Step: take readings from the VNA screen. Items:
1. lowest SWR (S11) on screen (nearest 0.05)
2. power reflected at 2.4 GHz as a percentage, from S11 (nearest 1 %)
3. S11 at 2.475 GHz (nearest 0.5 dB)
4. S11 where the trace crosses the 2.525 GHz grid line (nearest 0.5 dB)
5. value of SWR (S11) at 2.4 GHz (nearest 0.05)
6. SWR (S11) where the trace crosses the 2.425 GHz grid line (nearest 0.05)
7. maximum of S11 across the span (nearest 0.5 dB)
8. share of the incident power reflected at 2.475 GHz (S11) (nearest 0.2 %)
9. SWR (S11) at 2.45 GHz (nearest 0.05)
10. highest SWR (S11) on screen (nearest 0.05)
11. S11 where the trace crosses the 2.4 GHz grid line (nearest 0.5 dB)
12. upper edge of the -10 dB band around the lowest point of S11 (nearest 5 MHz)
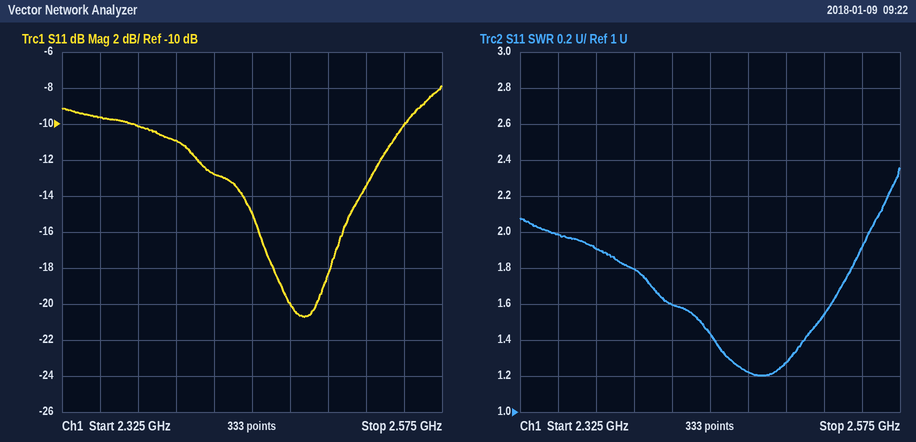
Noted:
1.20
8 %
-20.0 dB
-13.5 dB
1.80
1.60
-8.0 dB
1.0 %
1.45
2.35
-11.0 dB
2.550 GHz
